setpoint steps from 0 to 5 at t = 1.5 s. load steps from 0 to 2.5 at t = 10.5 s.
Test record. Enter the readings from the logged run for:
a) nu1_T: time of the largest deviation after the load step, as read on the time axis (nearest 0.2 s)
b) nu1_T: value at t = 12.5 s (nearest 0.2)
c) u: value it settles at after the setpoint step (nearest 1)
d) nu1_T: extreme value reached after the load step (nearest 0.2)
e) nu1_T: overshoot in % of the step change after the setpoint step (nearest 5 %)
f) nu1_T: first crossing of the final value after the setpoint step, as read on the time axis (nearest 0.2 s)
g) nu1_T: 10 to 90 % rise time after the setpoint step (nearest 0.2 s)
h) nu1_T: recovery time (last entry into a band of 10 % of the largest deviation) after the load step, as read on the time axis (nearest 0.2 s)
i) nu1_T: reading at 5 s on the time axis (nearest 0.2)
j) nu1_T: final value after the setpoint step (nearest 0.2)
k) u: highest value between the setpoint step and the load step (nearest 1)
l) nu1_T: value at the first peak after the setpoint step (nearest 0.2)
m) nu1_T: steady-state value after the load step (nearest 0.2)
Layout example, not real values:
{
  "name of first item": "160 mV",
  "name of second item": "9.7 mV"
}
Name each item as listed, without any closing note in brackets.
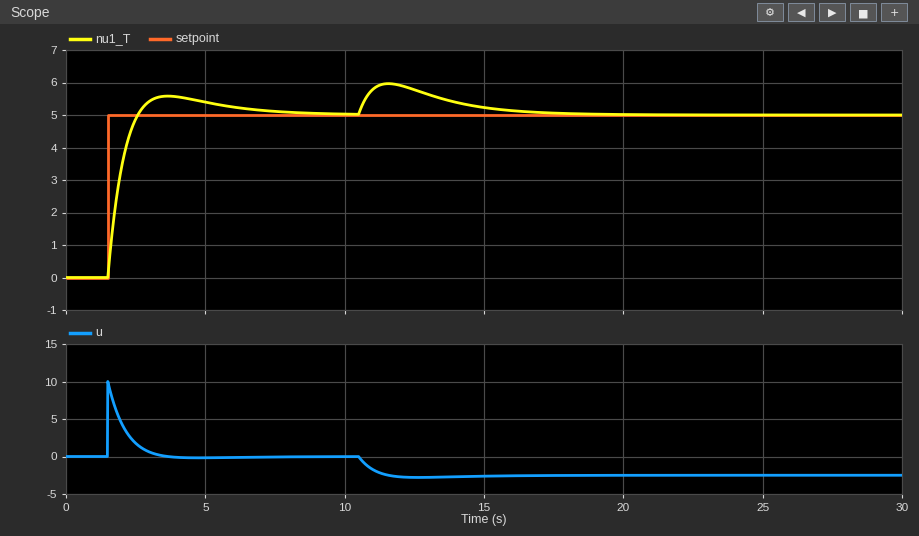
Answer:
{
  "nu1_T: time of the largest deviation after the load step, as read on the time axis": "11.6 s",
  "nu1_T: value at t = 12.5 s": "5.8",
  "u: value it settles at after the setpoint step": "0",
  "nu1_T: extreme value reached after the load step": "6.0",
  "nu1_T: overshoot in % of the step change after the setpoint step": "10 %",
  "nu1_T: first crossing of the final value after the setpoint step, as read on the time axis": "2.6 s",
  "nu1_T: 10 to 90 % rise time after the setpoint step": "0.8 s",
  "nu1_T: recovery time (last entry into a band of 10 % of the largest deviation) after the load step, as read on the time axis": "16.6 s",
  "nu1_T: reading at 5 s on the time axis": "5.4",
  "nu1_T: final value after the setpoint step": "5.0",
  "u: highest value between the setpoint step and the load step": "10",
  "nu1_T: value at the first peak after the setpoint step": "5.6",
  "nu1_T: steady-state value after the load step": "5.0"
}
